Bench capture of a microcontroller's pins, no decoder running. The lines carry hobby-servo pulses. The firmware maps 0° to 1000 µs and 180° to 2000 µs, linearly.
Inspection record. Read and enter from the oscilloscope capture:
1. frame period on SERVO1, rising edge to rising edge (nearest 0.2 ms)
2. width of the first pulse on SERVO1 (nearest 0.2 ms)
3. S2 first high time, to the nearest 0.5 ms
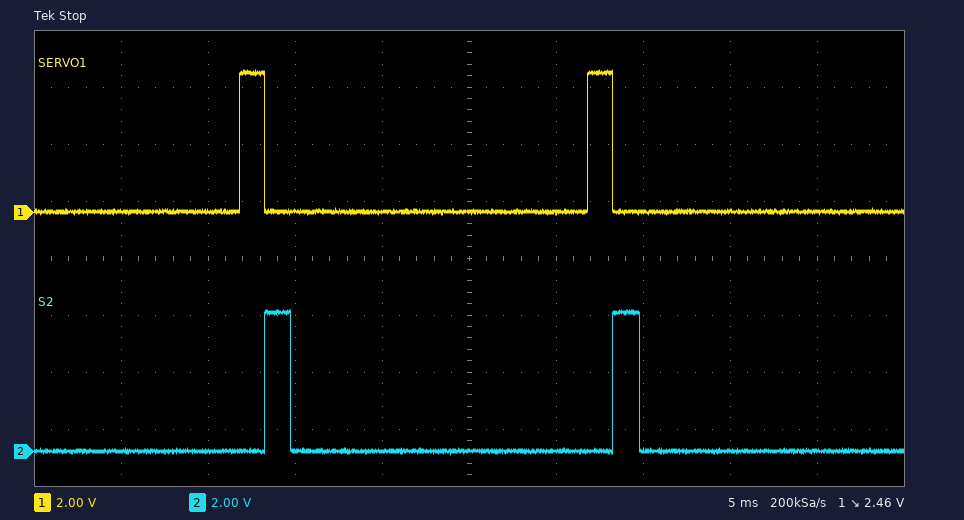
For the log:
20.0 ms
1.4 ms
1.5 ms
